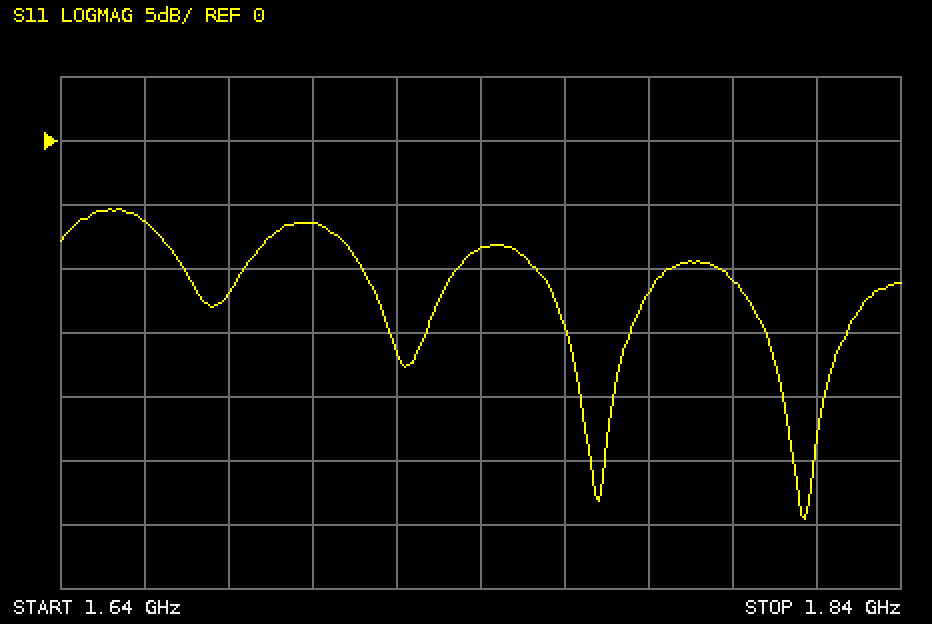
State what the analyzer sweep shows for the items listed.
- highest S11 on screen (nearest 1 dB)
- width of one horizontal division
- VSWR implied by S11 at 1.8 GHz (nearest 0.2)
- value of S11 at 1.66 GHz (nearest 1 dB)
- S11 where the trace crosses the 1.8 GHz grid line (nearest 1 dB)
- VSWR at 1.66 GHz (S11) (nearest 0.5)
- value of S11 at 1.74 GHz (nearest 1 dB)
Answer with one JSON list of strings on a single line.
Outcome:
["-5 dB", "20 MHz", "1.8", "-6 dB", "-11 dB", "3.0", "-8 dB"]
